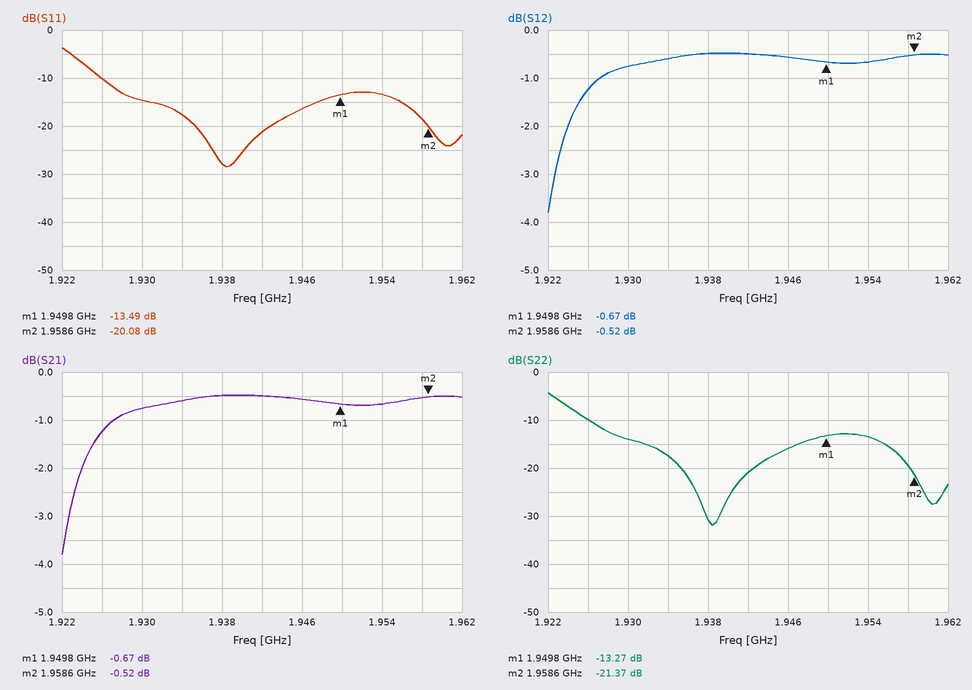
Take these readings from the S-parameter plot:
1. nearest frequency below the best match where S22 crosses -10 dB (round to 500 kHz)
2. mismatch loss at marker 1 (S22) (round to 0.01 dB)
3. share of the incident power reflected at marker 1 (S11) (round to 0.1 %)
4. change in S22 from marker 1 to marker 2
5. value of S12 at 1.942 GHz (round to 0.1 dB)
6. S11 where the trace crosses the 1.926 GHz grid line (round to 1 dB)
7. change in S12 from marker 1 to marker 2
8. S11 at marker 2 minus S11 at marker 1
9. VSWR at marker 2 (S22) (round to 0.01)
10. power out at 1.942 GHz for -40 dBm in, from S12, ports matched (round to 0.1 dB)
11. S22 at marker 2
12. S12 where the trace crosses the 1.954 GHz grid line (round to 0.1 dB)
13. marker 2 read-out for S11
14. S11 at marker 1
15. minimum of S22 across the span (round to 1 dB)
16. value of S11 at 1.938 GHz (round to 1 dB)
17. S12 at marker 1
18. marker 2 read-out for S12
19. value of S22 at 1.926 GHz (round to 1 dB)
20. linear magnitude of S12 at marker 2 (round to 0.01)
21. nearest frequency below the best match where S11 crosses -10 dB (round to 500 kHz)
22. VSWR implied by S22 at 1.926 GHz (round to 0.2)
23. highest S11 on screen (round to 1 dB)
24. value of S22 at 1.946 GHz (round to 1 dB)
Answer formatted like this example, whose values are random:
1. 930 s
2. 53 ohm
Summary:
1. 1.9260 GHz
2. 0.21 dB
3. 4.5 %
4. -8.10 dB
5. -0.5 dB
6. -10 dB
7. 0.15 dB
8. -6.59 dB
9. 1.19
10. -40.5 dBm
11. -21.37 dB
12. -0.7 dB
13. -20.08 dB
14. -13.49 dB
15. -32 dB
16. -28 dB
17. -0.67 dB
18. -0.52 dB
19. -10 dB
20. 0.94
21. 1.9260 GHz
22. 2.0
23. -4 dB
24. -16 dB
